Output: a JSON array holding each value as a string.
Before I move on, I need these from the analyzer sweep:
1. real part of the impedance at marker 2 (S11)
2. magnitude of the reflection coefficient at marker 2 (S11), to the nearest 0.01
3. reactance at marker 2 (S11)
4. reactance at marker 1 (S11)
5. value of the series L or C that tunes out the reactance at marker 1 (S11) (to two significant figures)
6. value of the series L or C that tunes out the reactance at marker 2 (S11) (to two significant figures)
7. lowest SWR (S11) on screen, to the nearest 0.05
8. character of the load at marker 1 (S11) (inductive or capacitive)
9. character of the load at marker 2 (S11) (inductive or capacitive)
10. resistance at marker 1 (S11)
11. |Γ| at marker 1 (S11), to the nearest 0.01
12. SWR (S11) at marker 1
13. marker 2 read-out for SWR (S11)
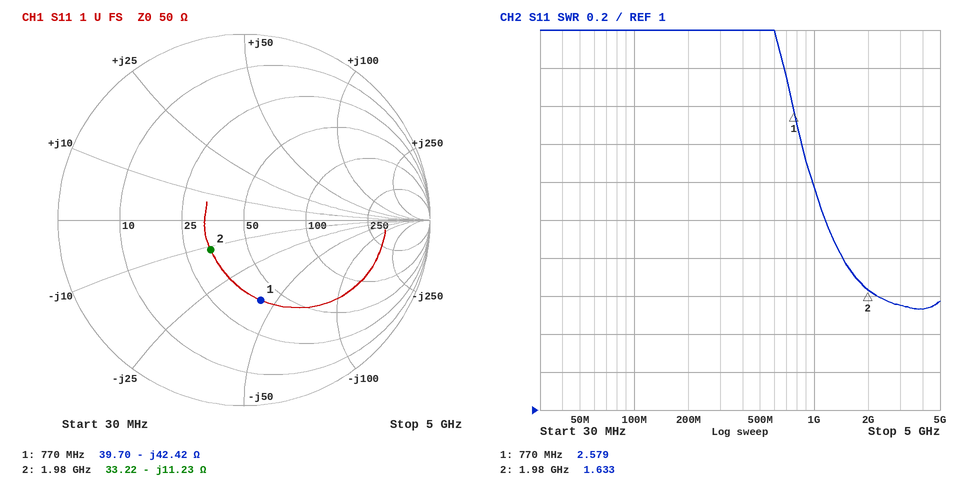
["33.22 Ω", "0.24", "-11.23 Ω", "-42.42 Ω", "8.8 nH", "900 pH", "1.55", "capacitive", "capacitive", "39.70 Ω", "0.44", "2.579", "1.633"]
